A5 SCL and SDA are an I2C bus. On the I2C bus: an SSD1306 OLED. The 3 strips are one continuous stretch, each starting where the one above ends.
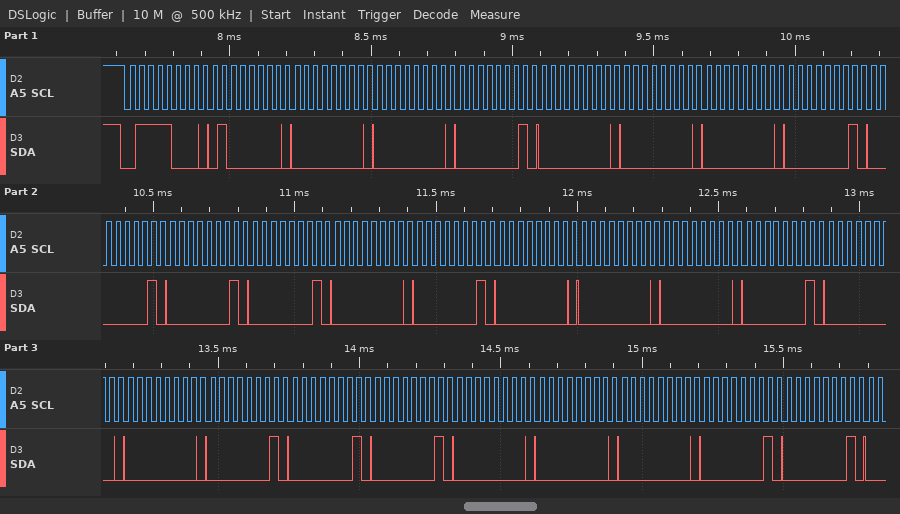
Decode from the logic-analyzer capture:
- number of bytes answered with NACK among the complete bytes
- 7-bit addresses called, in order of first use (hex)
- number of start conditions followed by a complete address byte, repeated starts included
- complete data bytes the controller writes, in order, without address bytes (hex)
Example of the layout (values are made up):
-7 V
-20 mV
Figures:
0
0x3C
1
40 00 00 01 00 00 00 01 01 01 01 00 01 00 00 00 01 00 00 01 01 01 00 00 00 01 01
